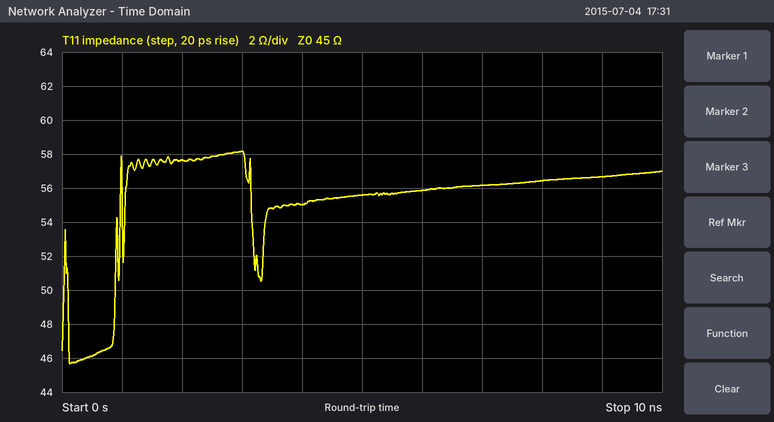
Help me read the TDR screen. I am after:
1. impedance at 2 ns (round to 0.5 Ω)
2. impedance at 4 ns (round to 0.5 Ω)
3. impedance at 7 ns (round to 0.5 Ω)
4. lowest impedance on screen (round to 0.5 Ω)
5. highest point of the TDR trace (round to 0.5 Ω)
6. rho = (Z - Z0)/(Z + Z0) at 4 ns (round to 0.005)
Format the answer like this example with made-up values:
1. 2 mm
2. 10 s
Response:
1. 57.5 Ω
2. 55.0 Ω
3. 56.0 Ω
4. 45.5 Ω
5. 58.0 Ω
6. +0.100
